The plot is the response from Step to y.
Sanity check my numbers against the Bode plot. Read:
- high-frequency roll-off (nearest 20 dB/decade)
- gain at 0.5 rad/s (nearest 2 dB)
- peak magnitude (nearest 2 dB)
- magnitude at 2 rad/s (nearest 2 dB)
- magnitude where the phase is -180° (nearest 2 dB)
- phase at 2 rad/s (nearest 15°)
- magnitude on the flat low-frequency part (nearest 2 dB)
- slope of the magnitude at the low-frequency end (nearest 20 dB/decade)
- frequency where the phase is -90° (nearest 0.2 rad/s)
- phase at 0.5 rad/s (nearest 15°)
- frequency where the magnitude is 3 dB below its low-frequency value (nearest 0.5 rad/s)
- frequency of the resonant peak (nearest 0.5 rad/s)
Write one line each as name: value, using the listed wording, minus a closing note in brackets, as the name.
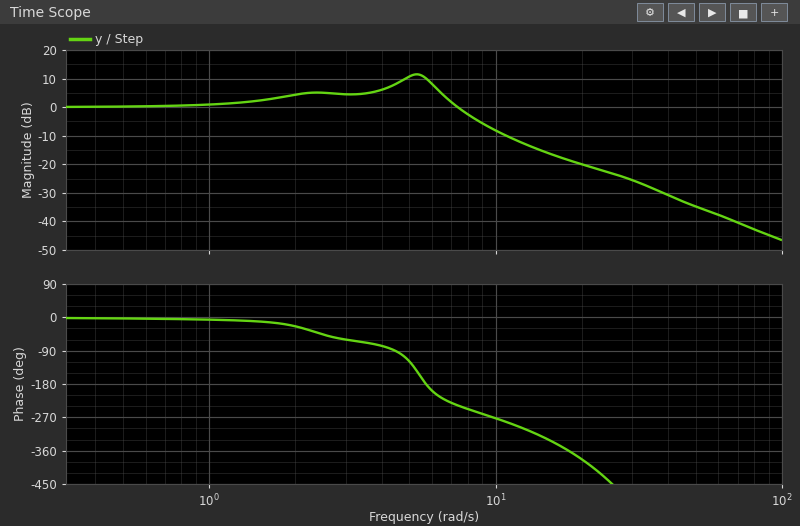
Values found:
high-frequency roll-off: -40 dB/decade
gain at 0.5 rad/s: 0 dB
peak magnitude: 12 dB
magnitude at 2 rad/s: 4 dB
magnitude where the phase is -180°: 10 dB
phase at 2 rad/s: -30°
magnitude on the flat low-frequency part: 0 dB
slope of the magnitude at the low-frequency end: 0 dB/decade
frequency where the phase is -90°: 4.4 rad/s
phase at 0.5 rad/s: 0°
frequency where the magnitude is 3 dB below its low-frequency value: 8.0 rad/s
frequency of the resonant peak: 5.5 rad/s
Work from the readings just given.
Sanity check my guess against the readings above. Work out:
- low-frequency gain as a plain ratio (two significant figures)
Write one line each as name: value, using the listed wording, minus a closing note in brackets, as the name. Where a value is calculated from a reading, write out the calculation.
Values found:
low-frequency gain as a plain ratio: 10^(0 / 20) = 1.0
